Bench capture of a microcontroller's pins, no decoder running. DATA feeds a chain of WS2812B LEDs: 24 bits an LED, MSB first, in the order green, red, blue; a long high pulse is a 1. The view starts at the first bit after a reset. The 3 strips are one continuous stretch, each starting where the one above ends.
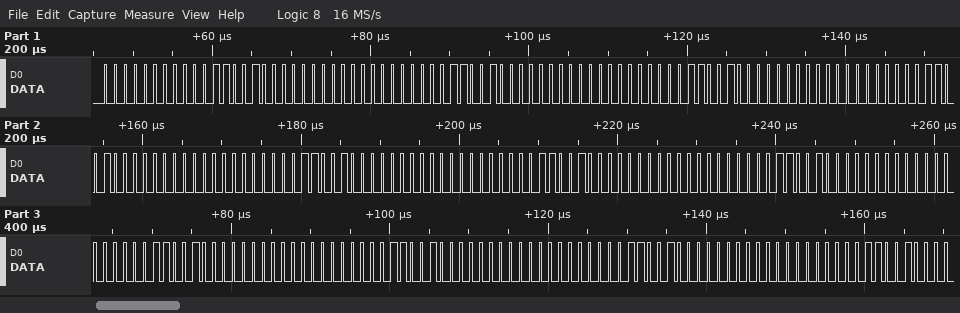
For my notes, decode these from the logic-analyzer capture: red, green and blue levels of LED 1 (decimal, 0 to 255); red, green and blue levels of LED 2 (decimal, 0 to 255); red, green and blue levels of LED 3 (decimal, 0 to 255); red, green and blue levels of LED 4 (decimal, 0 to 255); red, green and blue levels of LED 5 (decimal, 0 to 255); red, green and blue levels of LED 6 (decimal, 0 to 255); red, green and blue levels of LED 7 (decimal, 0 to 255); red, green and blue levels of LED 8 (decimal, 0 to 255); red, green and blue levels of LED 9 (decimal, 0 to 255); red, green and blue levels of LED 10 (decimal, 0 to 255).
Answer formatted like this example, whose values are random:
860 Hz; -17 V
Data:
25, 0, 0; 25, 0, 0; 25, 0, 0; 25, 0, 0; 25, 0, 0; 25, 0, 0; 25, 0, 0; 25, 0, 0; 25, 0, 0; 25, 0, 0
